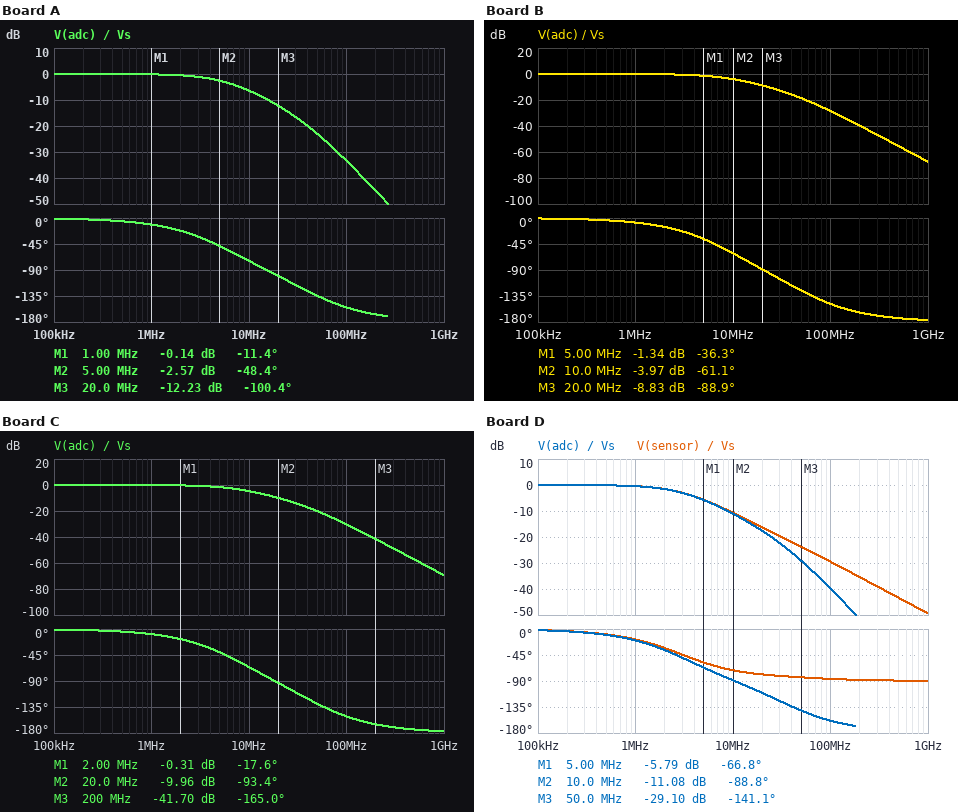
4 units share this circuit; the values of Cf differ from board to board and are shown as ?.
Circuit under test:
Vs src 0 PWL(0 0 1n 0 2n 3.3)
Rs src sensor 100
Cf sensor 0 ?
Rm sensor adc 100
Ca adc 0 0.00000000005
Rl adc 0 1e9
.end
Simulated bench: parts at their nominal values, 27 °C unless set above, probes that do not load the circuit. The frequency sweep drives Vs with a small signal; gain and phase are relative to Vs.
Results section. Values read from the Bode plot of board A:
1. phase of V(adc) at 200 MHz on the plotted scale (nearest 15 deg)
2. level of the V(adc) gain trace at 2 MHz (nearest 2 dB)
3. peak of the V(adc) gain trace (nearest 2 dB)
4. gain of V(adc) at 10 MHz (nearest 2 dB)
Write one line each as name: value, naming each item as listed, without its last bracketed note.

phase of V(adc) at 200 MHz on the plotted scale: -165 deg
level of the V(adc) gain trace at 2 MHz: 0 dB
peak of the V(adc) gain trace: 0 dB
gain of V(adc) at 10 MHz: -6 dB
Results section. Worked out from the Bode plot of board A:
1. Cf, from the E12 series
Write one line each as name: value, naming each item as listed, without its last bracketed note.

Cf, from the E12 series: 220 pF
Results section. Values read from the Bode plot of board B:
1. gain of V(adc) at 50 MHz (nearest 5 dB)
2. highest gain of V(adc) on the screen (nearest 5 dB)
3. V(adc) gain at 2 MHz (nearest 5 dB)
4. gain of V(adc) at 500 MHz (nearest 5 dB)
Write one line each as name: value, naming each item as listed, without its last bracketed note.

gain of V(adc) at 50 MHz: -20 dB
highest gain of V(adc) on the screen: 0 dB
V(adc) gain at 2 MHz: 0 dB
gain of V(adc) at 500 MHz: -55 dB
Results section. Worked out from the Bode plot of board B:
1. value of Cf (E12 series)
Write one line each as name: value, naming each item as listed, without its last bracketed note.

value of Cf: 120 pF
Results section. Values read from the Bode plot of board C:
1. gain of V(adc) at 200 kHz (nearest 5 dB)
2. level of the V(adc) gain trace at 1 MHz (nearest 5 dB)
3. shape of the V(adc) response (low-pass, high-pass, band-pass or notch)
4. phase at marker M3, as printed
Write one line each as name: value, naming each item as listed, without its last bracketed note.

gain of V(adc) at 200 kHz: 0 dB
level of the V(adc) gain trace at 1 MHz: 0 dB
shape of the V(adc) response: low-pass
phase at marker M3, as printed: -165.0 deg
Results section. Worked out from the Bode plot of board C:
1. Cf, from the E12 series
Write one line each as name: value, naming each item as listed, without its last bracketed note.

Cf, from the E12 series: 150 pF
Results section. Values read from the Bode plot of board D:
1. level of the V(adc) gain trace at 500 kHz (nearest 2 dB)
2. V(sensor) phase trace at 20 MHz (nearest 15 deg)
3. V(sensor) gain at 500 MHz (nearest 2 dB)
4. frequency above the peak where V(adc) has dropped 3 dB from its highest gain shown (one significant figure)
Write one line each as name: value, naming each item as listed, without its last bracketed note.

level of the V(adc) gain trace at 500 kHz: 0 dB
V(sensor) phase trace at 20 MHz: -75 deg
V(sensor) gain at 500 MHz: -44 dB
frequency above the peak where V(adc) has dropped 3 dB from its highest gain shown: 3 MHz
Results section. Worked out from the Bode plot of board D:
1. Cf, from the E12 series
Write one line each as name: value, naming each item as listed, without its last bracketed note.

Cf, from the E12 series: 470 pF
